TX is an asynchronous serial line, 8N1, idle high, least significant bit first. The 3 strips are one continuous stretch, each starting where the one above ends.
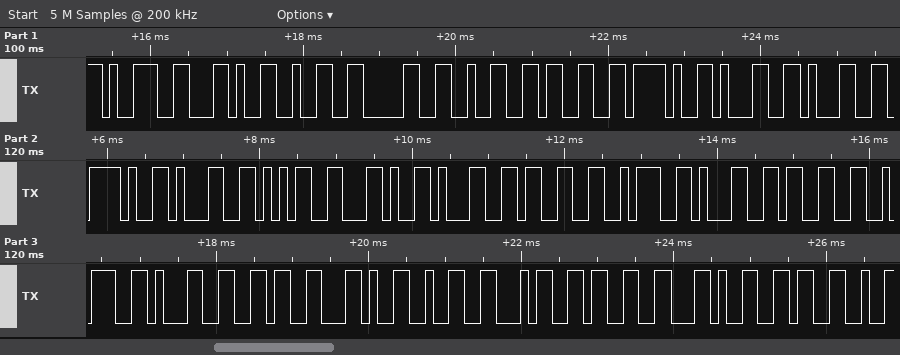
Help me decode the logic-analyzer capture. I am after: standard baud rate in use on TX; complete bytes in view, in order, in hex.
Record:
9600 baud
39 2C 32 30 32 33 2F 31 31 2F 31 35 2C 31 33 3A 31 33 3A 31 36 2C 32 34 33 2C 36
